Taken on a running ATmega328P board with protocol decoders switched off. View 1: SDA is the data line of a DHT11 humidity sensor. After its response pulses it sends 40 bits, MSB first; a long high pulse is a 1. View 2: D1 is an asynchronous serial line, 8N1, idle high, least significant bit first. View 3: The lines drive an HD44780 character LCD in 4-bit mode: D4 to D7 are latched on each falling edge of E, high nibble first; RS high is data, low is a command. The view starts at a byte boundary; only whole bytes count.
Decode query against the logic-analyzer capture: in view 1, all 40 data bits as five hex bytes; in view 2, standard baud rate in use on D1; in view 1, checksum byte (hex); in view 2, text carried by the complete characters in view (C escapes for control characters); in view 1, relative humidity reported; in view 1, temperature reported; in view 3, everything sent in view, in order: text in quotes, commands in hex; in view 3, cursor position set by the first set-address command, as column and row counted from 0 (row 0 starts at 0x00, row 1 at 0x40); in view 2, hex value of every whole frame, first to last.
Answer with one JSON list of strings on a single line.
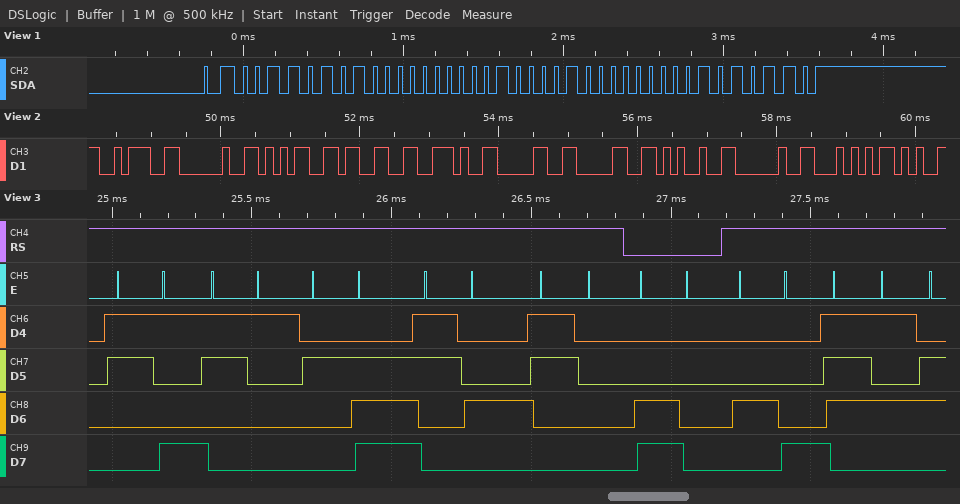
["35 00 21 00 56", "9600 baud", "0x56", "\": 53.00% T\"", "53 %", "33.0 °C", "\"91.40\" 0xC0 \"Hu\"", "column 0, row 1", "3A 20 35 33 2E 30 30 25 20 54"]
